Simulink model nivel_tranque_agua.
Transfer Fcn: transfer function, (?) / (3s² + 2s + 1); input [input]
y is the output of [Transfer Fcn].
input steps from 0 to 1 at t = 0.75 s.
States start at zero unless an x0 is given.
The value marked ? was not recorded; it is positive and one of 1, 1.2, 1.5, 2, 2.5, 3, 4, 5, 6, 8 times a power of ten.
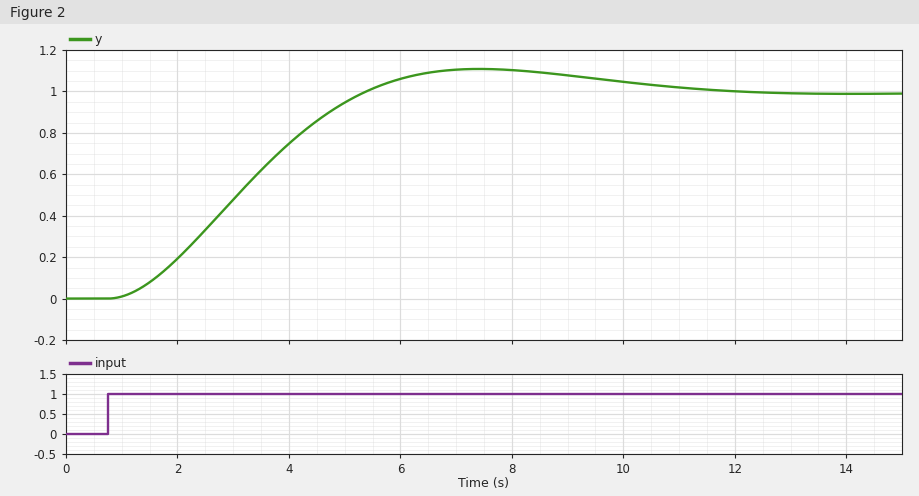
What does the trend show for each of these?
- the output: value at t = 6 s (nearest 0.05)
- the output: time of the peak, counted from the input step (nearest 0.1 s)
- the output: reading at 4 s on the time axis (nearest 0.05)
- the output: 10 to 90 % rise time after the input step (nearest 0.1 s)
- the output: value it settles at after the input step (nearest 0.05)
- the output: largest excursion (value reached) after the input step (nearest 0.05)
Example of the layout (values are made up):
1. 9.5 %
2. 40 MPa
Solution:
1. 1.05
2. 6.7 s
3. 0.75
4. 3.1 s
5. 1.00
6. 1.10
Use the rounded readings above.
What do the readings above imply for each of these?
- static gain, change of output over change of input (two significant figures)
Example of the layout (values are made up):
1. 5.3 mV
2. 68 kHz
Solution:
1. 1.0
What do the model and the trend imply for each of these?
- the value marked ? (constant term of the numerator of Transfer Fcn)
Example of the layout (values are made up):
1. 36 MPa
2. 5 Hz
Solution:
1. 1
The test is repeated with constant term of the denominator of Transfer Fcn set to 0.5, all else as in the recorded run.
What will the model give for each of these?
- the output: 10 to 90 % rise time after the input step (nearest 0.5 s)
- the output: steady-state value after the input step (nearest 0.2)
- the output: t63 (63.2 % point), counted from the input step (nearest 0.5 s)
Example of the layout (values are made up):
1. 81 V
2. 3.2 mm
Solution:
1. 6.0 s
2. 2.0
3. 4.5 s
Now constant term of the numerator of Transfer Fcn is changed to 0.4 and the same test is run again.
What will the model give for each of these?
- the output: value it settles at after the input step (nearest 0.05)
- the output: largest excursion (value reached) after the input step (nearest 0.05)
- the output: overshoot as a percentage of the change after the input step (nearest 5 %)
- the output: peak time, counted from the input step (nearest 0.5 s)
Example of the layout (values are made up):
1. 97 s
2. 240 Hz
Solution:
1. 0.40
2. 0.45
3. 10 %
4. 6.5 s
